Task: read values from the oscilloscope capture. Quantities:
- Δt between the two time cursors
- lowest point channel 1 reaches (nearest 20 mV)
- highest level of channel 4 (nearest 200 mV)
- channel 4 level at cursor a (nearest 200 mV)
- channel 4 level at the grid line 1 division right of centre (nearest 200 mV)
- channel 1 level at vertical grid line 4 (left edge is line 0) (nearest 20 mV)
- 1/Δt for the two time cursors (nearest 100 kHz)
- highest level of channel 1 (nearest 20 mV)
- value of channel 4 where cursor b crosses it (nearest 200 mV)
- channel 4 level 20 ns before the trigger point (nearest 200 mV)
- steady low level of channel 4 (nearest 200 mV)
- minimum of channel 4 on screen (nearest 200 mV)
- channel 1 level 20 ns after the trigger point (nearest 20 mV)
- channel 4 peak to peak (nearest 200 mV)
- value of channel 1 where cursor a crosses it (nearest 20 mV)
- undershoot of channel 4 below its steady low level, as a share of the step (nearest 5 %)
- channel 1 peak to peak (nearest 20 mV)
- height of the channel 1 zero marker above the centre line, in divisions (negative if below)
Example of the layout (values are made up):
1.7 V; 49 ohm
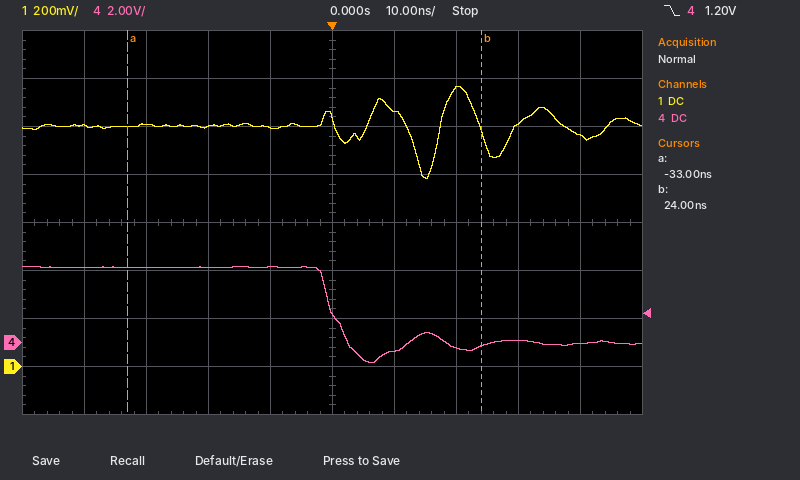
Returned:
57 ns; 780 mV; 3.2 V; 3.2 V; -400 mV; 1.00 V; 17.5 MHz; 1.16 V; -200 mV; 3.2 V; 0.0 V; -800 mV; 1.16 V; 4.0 V; 1.00 V; 25 %; 380 mV; -3.0 div
